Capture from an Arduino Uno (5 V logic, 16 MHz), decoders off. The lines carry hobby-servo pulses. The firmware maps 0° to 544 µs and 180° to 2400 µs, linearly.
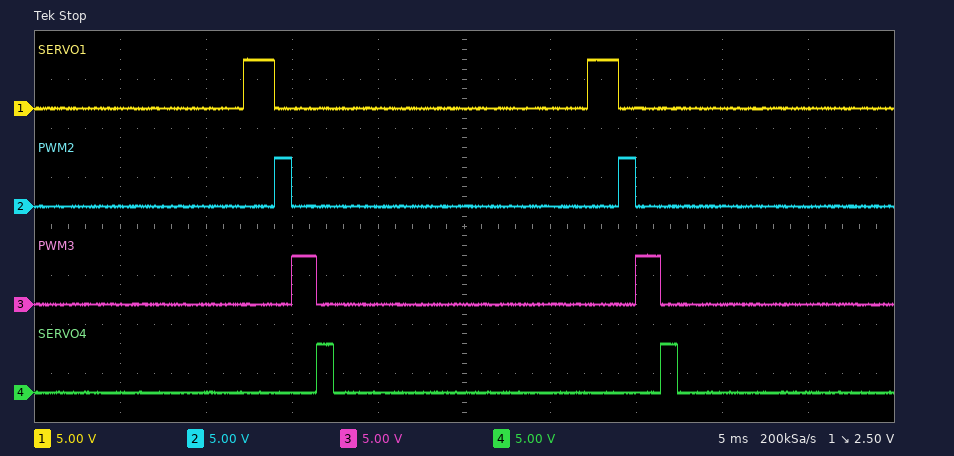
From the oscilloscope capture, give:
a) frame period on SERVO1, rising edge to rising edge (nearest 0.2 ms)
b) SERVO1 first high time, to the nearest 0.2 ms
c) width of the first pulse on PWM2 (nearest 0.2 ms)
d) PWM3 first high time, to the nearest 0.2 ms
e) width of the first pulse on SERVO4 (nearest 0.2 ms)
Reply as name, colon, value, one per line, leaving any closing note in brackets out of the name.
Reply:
frame period on SERVO1, rising edge to rising edge: 20.0 ms
SERVO1 first high time, to the nearest 0.2 ms: 1.8 ms
width of the first pulse on PWM2: 1.0 ms
PWM3 first high time, to the nearest 0.2 ms: 1.4 ms
width of the first pulse on SERVO4: 1.0 ms
